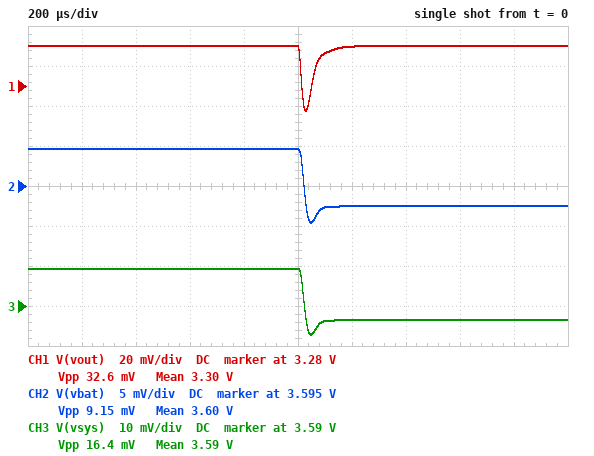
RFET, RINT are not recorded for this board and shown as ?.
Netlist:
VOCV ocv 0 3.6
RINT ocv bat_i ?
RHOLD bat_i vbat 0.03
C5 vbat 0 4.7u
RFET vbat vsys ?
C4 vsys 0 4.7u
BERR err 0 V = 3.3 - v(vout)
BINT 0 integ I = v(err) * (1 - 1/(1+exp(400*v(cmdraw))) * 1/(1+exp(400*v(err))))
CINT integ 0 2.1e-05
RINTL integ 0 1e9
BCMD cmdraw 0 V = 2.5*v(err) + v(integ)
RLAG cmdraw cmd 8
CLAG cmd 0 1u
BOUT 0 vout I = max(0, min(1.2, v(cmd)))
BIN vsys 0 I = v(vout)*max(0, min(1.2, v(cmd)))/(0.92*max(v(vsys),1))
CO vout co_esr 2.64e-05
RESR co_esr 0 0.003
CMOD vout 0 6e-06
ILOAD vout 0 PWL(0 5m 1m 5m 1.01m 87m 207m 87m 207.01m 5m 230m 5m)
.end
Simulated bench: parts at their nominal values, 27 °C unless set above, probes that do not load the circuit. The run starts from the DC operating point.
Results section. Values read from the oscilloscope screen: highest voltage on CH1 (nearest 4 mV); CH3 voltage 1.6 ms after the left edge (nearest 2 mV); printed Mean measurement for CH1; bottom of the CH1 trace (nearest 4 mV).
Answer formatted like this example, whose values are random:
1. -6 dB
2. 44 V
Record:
1. 3.300 V
2. 3.586 V
3. 3.30 V
4. 3.268 V
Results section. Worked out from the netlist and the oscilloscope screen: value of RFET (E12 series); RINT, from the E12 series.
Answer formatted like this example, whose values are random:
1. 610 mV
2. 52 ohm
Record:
1. 0.068 Ω
2. 0.056 Ω
